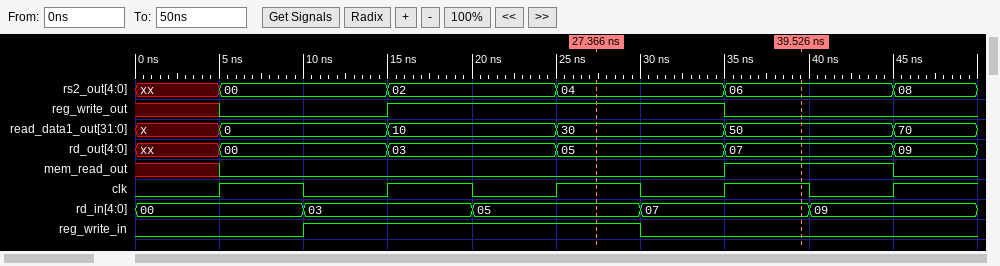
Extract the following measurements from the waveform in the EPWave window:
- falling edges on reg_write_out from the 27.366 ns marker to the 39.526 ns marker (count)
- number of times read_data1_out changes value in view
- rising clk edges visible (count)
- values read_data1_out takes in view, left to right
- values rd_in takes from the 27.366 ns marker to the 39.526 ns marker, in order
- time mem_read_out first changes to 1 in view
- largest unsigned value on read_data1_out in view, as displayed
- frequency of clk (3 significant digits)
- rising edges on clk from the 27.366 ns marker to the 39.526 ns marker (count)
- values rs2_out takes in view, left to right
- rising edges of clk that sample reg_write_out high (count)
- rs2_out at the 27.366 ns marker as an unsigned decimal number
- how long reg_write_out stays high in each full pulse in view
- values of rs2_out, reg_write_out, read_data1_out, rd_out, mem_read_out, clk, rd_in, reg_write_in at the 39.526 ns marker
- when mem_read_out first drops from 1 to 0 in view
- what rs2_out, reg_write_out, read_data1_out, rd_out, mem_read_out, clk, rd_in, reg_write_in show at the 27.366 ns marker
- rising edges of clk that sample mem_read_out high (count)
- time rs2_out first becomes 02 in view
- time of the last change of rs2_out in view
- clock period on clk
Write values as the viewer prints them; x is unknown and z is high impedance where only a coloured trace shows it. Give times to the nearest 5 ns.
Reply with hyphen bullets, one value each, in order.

- 1
- 5
- 5
- x, 0, 10, 30, 50, 70
- 05, 07
- 35 ns
- 70
- 100 MHz
- 1
- xx, 00, 02, 04, 06, 08
- 2
- 4
- 20 ns
- rs2_out=06, reg_write_out=0, read_data1_out=50, rd_out=07, mem_read_out=1, clk=1, rd_in=07, reg_write_in=0
- 45 ns
- rs2_out=04, reg_write_out=1, read_data1_out=30, rd_out=05, mem_read_out=0, clk=1, rd_in=05, reg_write_in=1
- 1
- 15 ns
- 45 ns
- 10 ns
